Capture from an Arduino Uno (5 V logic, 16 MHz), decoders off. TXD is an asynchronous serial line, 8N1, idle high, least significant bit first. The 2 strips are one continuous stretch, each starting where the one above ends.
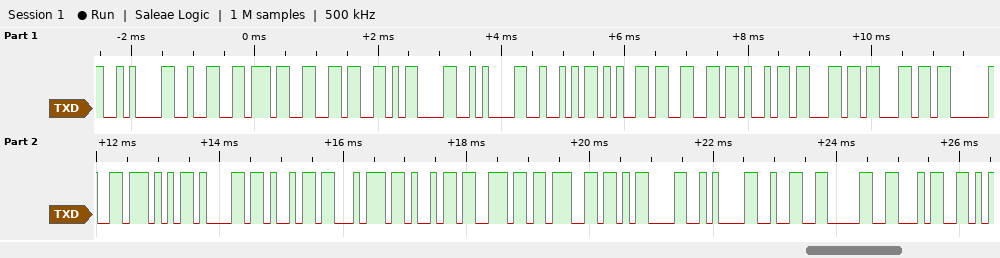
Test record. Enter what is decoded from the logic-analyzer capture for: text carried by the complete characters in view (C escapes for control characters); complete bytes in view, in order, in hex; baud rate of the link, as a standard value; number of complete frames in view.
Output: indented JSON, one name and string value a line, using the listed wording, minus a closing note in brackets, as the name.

{
  "text carried by the complete characters in view": "\"\\n276\\r\\nRefill Waiting\\r\\n204\"",
  "complete bytes in view, in order, in hex": "0A 32 37 36 0D 0A 52 65 66 69 6C 6C 20 57 61 69 74 69 6E 67 0D 0A 32 30 34",
  "baud rate of the link, as a standard value": "9600 baud",
  "number of complete frames in view": "25"
}
